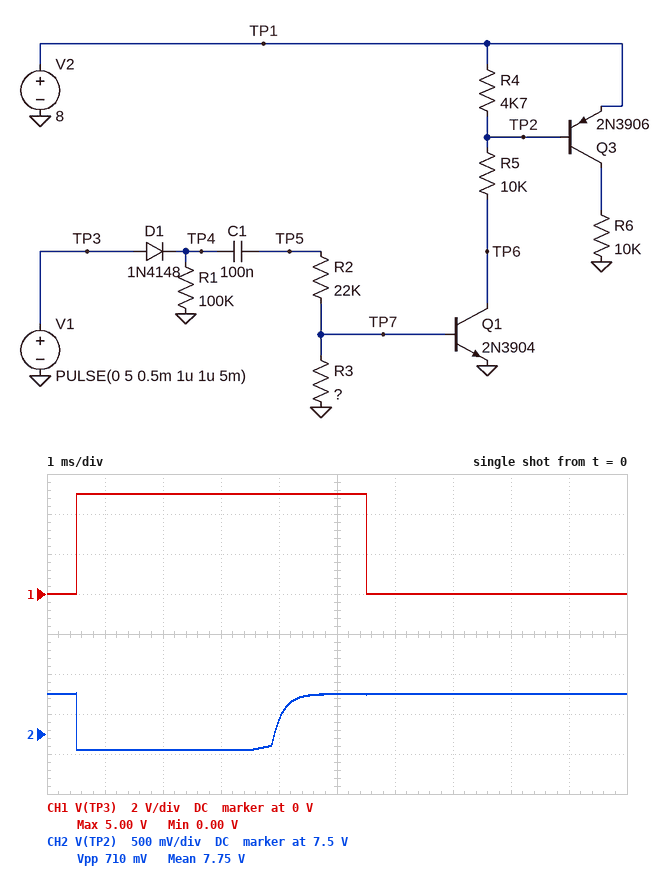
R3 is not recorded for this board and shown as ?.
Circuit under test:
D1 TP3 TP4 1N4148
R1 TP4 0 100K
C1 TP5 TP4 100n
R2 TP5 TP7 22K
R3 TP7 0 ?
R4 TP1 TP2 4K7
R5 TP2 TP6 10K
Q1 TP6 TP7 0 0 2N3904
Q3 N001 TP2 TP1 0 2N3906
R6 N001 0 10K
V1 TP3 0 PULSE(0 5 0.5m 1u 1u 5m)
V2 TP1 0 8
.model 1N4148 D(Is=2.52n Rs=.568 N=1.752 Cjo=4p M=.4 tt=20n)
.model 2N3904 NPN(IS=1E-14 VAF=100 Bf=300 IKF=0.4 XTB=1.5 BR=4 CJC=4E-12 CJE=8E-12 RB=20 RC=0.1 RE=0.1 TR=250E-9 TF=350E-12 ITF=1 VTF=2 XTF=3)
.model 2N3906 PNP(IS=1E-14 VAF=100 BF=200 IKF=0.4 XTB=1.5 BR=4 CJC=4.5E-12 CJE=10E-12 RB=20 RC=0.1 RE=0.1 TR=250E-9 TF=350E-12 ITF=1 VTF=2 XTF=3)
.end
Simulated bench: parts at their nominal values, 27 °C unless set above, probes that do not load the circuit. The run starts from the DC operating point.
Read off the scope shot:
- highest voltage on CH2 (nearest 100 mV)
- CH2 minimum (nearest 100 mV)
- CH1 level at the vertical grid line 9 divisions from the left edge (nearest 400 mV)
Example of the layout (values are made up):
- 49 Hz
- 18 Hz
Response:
- 8.0 V
- 7.3 V
- 0 V
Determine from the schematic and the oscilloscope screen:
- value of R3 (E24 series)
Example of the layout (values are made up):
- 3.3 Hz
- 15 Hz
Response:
- 15 kΩ
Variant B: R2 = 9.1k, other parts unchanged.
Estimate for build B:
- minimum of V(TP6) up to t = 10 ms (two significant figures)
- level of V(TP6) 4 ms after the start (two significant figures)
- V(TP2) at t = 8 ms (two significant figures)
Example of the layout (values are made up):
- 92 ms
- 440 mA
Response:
- 15 mV
- 8.0 V
- 8.0 V
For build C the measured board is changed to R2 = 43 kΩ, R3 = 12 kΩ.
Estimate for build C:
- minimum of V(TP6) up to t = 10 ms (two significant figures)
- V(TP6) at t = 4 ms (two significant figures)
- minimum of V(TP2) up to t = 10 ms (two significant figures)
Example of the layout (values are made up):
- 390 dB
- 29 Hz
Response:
- 50 mV
- 7.9 V
- 7.3 V
